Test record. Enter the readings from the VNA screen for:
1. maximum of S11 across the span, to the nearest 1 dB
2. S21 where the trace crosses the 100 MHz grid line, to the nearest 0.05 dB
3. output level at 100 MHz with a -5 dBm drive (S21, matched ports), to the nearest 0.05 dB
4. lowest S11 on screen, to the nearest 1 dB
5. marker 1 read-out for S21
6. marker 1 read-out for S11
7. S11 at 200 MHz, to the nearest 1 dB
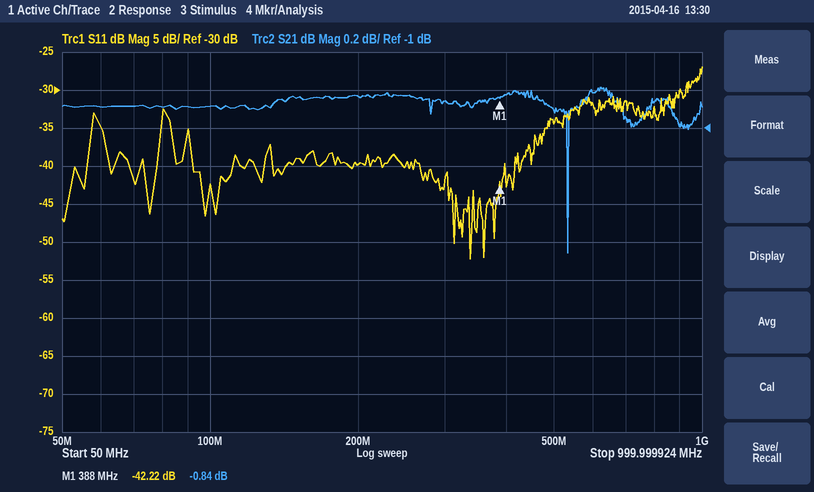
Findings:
-27 dB
-0.90 dB
-5.90 dBm
-52 dB
-0.84 dB
-42.22 dB
-40 dB
